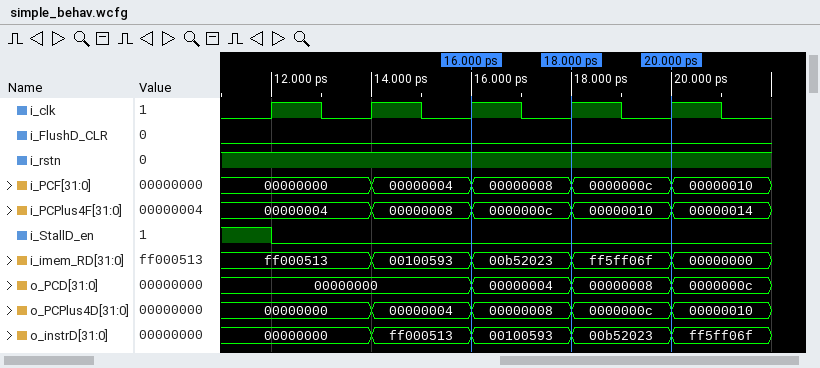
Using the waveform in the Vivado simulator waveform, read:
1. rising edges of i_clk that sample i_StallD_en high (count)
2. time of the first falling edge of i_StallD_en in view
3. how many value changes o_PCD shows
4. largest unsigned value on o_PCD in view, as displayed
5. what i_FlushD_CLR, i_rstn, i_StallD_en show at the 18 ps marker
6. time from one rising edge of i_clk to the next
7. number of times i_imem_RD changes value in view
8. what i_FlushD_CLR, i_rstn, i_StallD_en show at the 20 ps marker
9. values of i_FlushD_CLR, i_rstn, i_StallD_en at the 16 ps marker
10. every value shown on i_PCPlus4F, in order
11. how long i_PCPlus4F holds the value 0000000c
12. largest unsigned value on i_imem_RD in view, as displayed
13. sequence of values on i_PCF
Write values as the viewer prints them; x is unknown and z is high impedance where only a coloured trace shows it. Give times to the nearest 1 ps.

1
12 ps
3
0000000c
i_FlushD_CLR=0, i_rstn=1, i_StallD_en=0
2 ps
4
i_FlushD_CLR=0, i_rstn=1, i_StallD_en=0
i_FlushD_CLR=0, i_rstn=1, i_StallD_en=0
00000004, 00000008, 0000000c, 00000010, 00000014
2 ps
ff5ff06f
00000000, 00000004, 00000008, 0000000c, 00000010
